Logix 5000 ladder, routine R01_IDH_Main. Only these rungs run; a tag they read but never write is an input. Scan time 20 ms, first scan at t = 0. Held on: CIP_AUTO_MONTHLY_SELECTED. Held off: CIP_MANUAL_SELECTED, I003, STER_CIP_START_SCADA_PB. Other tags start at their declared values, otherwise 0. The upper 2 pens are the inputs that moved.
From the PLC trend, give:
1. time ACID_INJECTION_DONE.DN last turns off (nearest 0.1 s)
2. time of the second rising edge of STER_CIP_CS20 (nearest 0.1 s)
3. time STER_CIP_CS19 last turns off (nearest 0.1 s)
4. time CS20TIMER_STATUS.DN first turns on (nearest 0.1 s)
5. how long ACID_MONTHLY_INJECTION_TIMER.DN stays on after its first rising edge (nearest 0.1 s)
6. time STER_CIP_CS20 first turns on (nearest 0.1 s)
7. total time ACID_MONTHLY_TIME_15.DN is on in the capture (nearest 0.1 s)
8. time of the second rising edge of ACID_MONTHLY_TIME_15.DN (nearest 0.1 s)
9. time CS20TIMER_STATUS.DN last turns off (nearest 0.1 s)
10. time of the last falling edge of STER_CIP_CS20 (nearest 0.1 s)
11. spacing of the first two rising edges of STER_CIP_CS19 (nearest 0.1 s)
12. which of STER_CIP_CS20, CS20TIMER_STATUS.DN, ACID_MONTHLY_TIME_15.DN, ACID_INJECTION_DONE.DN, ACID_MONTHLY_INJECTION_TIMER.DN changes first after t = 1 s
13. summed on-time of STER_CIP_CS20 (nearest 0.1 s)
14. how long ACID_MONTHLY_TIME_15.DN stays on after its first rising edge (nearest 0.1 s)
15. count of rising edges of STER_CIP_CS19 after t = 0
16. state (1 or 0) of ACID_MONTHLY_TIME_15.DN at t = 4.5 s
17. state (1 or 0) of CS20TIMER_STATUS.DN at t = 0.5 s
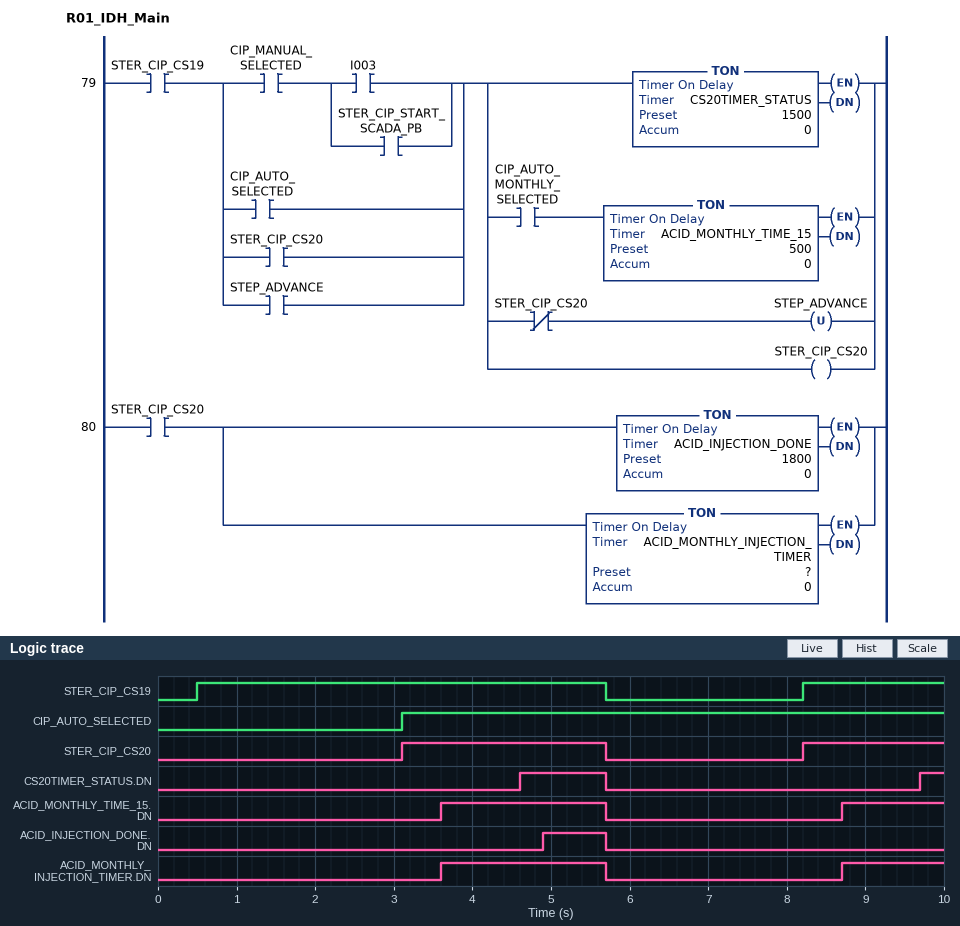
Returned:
5.7 s
8.2 s
5.7 s
4.6 s
2.1 s
3.1 s
3.4 s
8.7 s
5.7 s
5.7 s
7.7 s
STER_CIP_CS20
4.4 s
2.1 s
2
1
0
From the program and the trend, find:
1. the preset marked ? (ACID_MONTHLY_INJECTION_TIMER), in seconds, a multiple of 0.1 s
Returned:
0.5 s
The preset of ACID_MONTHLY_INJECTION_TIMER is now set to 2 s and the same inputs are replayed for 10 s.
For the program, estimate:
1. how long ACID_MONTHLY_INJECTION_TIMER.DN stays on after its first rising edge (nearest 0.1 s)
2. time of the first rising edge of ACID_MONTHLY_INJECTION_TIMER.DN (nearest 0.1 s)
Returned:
0.6 s
5.1 s
